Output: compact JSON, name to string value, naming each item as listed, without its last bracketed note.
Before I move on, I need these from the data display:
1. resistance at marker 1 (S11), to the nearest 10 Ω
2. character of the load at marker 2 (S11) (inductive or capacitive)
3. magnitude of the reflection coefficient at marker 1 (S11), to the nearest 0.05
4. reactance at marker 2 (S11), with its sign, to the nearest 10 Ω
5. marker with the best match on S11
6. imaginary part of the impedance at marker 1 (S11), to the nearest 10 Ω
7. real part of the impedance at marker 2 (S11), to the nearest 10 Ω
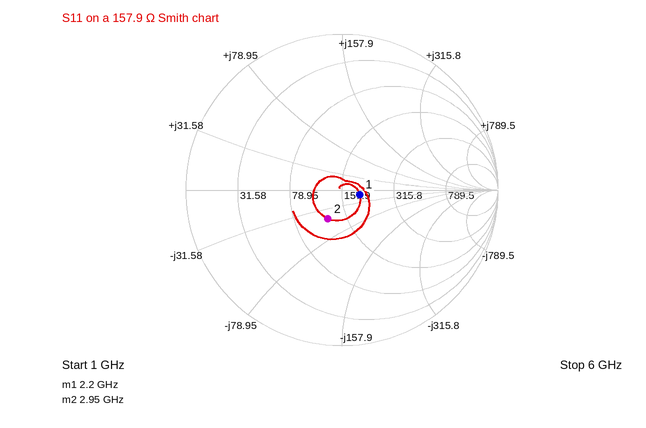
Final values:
{"resistance at marker 1 (S11), to the nearest 10 Ω": "200 Ω", "character of the load at marker 2 (S11)": "capacitive", "magnitude of the reflection coefficient at marker 1 (S11), to the nearest 0.05": "0.10", "reactance at marker 2 (S11), with its sign, to the nearest 10 Ω": "-50 Ω", "marker with the best match on S11": "marker 1", "imaginary part of the impedance at marker 1 (S11), to the nearest 10 Ω": "-10 Ω", "real part of the impedance at marker 2 (S11), to the nearest 10 Ω": "120 Ω"}
